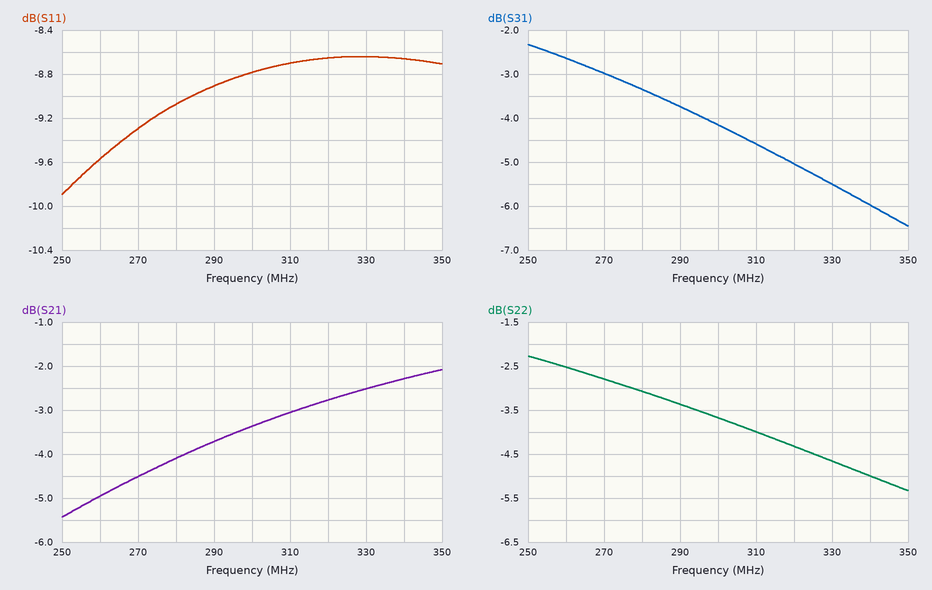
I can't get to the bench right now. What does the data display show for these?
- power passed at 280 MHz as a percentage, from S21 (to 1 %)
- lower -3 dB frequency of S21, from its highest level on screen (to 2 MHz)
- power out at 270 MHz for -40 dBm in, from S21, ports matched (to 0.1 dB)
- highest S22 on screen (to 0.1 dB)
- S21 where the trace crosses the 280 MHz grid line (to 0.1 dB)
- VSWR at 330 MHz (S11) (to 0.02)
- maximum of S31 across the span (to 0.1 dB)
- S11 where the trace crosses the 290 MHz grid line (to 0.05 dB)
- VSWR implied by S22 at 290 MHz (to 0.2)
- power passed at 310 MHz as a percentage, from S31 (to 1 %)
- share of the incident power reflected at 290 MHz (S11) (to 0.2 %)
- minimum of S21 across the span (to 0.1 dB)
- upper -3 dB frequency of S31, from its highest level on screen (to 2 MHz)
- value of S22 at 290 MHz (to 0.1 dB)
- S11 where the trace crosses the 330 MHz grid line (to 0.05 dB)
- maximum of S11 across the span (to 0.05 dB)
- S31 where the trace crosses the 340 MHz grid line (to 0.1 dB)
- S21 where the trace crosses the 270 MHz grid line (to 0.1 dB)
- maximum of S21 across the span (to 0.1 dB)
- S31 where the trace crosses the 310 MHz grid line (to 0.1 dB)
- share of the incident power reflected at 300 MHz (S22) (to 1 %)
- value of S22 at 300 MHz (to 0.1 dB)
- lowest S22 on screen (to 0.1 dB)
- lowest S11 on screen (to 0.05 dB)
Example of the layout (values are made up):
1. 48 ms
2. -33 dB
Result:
1. 39 %
2. 258 MHz
3. -44.5 dBm
4. -2.3 dB
5. -4.1 dB
6. 2.18
7. -2.3 dB
8. -8.90 dB
9. 5.2
10. 35 %
11. 12.8 %
12. -5.4 dB
13. 326 MHz
14. -3.4 dB
15. -8.65 dB
16. -8.65 dB
17. -6.0 dB
18. -4.5 dB
19. -2.1 dB
20. -4.6 dB
21. 43 %
22. -3.7 dB
23. -5.3 dB
24. -9.90 dB
